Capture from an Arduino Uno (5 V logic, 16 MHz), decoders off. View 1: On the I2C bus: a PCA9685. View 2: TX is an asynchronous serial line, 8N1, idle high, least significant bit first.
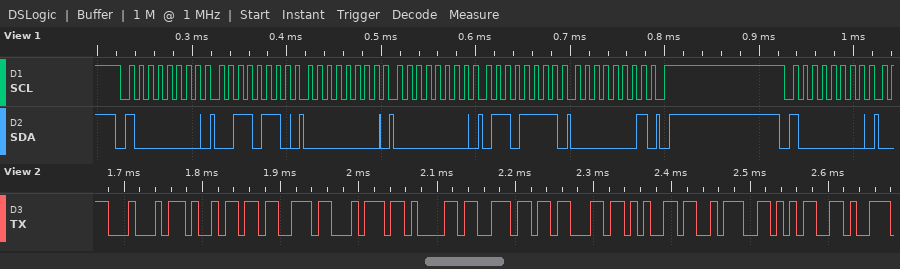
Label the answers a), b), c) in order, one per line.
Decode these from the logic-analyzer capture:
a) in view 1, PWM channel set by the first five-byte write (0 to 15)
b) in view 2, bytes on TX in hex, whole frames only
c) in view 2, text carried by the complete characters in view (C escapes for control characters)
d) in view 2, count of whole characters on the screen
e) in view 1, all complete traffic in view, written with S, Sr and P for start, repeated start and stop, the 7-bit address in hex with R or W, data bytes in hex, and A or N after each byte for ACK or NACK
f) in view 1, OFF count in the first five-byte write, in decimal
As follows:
a) 12
b) 44 69 73 74 61 6E 63 65 3A 35
c) "Distance:5"
d) 10
e) S 40W A 36 A 00 A 00 A 6F A 01 A P S 40W A
f) 367
